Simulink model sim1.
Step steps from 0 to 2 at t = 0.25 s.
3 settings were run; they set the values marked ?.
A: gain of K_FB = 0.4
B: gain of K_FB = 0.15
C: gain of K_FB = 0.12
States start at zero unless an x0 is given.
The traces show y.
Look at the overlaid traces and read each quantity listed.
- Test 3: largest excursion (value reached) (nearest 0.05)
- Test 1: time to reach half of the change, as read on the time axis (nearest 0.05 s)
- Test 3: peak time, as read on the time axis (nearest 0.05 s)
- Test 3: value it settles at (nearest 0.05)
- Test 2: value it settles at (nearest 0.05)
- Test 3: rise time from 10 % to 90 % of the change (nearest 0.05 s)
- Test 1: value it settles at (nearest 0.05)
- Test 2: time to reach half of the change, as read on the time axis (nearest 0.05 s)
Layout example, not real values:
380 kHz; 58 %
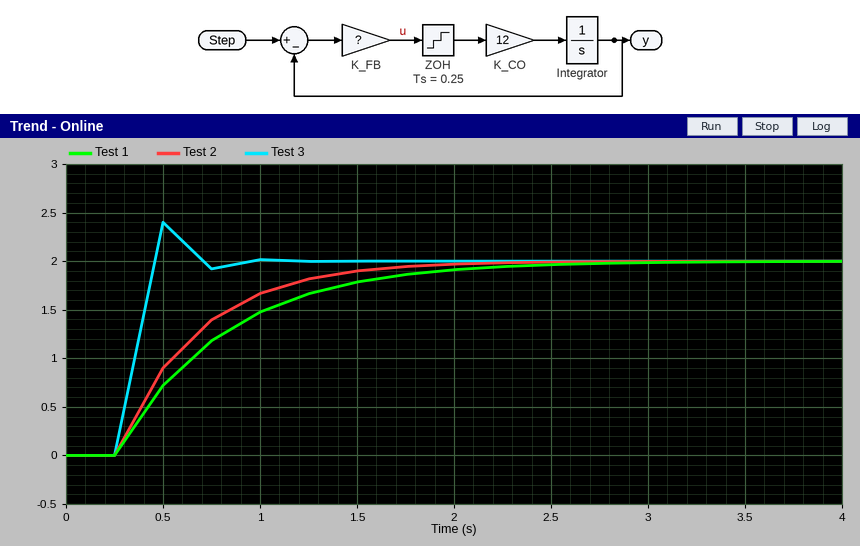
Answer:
2.40; 0.65 s; 0.50 s; 2.00; 2.00; 0.15 s; 2.00; 0.55 s
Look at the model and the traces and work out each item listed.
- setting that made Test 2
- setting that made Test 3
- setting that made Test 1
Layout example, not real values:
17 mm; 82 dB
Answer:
B; A; C
